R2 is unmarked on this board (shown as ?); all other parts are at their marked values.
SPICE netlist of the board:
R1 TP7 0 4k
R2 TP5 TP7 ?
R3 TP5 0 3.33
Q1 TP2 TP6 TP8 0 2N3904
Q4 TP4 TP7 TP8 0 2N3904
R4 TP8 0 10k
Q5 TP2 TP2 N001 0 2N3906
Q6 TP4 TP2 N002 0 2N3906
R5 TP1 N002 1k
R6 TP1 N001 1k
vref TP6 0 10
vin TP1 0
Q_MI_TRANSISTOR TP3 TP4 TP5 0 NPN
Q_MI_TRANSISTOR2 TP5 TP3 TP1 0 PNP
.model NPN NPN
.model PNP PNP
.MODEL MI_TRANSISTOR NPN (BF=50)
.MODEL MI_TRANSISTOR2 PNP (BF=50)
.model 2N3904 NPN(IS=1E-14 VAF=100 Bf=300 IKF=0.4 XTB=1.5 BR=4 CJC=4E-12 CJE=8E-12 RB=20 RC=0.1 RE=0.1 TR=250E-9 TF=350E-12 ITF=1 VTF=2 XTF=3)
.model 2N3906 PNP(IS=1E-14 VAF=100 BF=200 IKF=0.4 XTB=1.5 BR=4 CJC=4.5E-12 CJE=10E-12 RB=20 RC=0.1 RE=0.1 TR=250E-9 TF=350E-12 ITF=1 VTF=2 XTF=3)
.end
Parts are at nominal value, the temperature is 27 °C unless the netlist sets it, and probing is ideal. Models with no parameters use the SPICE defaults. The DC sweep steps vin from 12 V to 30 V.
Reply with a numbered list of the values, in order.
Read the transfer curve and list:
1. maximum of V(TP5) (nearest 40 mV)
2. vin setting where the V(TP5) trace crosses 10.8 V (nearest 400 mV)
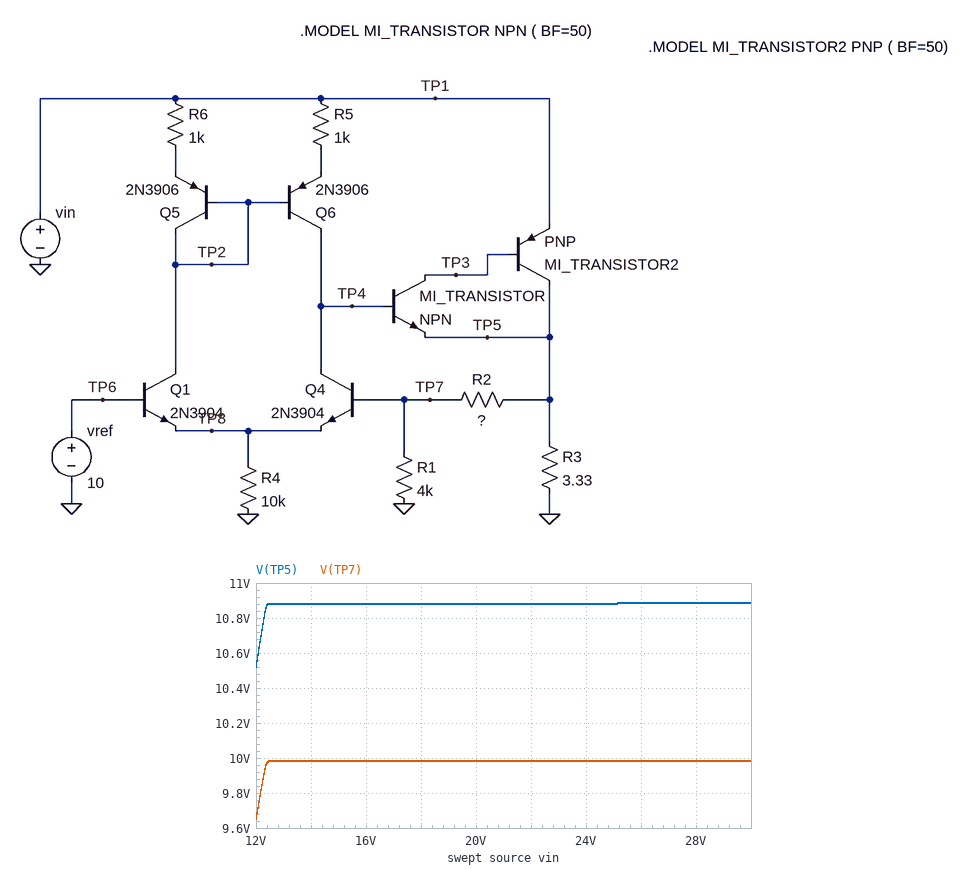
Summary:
1. 10.88 V
2. 12.4 V
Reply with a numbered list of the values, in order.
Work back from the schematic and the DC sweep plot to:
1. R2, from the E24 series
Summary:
1. 360 Ω
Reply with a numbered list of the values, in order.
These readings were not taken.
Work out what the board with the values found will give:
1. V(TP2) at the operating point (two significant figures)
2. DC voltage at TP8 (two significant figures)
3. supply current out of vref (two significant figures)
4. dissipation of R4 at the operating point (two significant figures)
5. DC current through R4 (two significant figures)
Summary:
1. 9.3 V
2. 9.3 V
3. 930 µA
4. 8.6 mW
5. 930 µA
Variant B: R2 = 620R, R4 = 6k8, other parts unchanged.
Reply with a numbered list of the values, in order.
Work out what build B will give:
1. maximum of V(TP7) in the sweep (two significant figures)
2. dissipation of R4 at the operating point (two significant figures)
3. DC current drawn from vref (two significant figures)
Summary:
1. 10 V
2. 13 mW
3. 1.4 mA
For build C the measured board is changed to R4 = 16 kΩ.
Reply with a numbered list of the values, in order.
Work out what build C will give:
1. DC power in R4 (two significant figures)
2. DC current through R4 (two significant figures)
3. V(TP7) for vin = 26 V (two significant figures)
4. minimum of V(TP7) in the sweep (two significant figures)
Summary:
1. 5.4 mW
2. 580 µA
3. 10 V
4. 9.8 V
